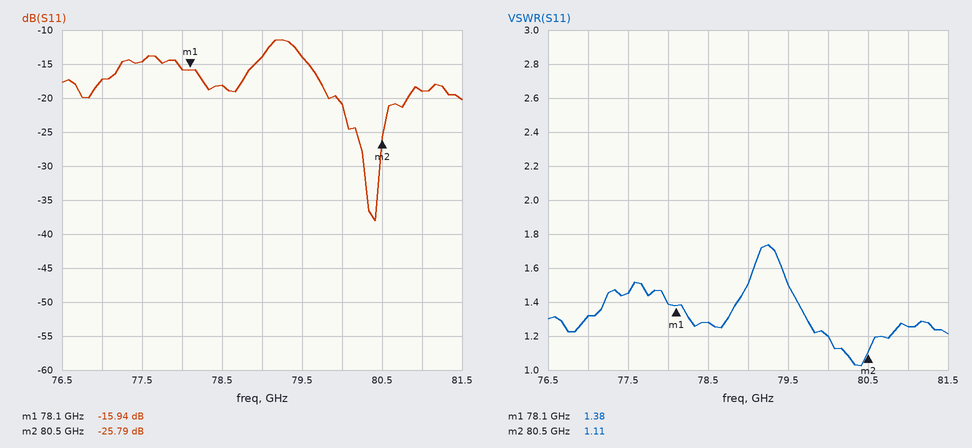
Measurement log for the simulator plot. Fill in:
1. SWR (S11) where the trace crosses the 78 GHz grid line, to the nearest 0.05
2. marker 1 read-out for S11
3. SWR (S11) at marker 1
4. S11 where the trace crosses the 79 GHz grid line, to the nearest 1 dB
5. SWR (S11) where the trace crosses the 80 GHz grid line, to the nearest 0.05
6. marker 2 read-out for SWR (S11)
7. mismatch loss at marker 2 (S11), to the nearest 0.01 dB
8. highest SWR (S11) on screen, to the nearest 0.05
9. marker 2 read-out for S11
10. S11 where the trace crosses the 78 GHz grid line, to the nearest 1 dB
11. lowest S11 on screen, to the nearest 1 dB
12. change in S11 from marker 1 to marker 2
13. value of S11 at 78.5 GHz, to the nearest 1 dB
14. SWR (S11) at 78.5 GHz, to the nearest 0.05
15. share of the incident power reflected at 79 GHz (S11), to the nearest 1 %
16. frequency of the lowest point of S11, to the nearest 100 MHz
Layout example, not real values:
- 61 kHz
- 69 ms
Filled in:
- 1.40
- -15.94 dB
- 1.38
- -14 dB
- 1.20
- 1.11
- 0.01 dB
- 1.75
- -25.79 dB
- -16 dB
- -38 dB
- -9.85 dB
- -18 dB
- 1.30
- 4 %
- 80.4 GHz
